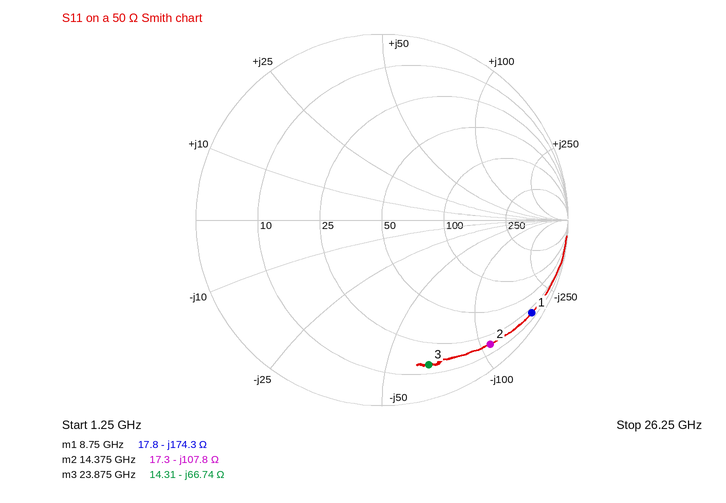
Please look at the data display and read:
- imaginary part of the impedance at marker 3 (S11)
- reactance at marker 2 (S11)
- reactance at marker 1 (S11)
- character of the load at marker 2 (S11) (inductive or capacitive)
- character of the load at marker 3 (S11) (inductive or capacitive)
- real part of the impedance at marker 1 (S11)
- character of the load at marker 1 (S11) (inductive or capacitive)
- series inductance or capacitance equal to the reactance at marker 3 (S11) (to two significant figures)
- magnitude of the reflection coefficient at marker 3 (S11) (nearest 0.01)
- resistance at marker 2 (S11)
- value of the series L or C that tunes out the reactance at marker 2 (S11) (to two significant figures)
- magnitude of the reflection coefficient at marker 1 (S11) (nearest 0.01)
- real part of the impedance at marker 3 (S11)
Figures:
-66.74 Ω
-107.8 Ω
-174.3 Ω
capacitive
capacitive
17.8 Ω
capacitive
100 fF
0.82
17.3 Ω
1.2 nH
0.95
14.31 Ω
